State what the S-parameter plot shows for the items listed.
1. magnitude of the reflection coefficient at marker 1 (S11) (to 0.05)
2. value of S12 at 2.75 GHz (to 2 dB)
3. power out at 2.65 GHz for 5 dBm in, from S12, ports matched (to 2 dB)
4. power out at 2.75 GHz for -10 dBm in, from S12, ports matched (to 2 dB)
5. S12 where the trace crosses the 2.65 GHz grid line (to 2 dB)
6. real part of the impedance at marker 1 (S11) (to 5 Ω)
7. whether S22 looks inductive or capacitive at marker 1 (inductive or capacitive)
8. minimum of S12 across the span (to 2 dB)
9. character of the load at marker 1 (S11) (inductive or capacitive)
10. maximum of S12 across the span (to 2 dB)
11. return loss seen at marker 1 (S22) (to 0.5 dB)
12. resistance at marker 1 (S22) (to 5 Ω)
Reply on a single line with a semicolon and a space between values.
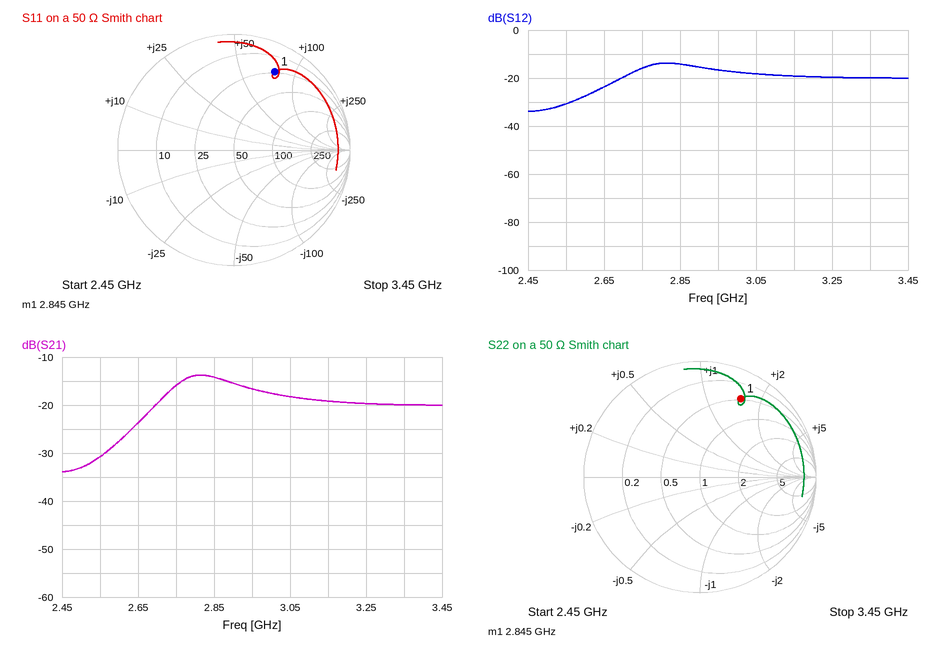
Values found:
0.75; -16 dB; -18 dBm; -26 dBm; -24 dB; 25 Ω; inductive; -34 dB; inductive; -14 dB; 2.5 dB; 25 Ω
